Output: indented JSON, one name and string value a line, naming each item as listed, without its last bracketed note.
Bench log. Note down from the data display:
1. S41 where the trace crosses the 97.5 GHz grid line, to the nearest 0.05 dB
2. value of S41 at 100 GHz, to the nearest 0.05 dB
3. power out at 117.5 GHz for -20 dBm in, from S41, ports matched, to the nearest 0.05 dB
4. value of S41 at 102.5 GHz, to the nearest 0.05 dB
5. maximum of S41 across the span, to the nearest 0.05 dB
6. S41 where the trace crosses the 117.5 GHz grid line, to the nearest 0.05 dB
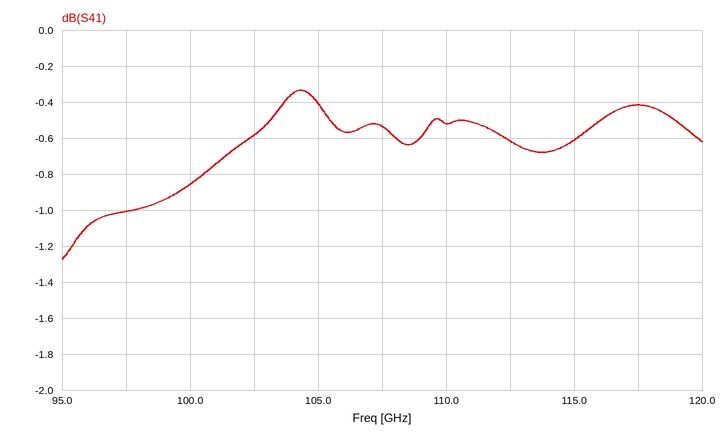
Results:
{
  "S41 where the trace crosses the 97.5 GHz grid line, to the nearest 0.05 dB": "-1.00 dB",
  "value of S41 at 100 GHz, to the nearest 0.05 dB": "-0.85 dB",
  "power out at 117.5 GHz for -20 dBm in, from S41, ports matched, to the nearest 0.05 dB": "-20.40 dBm",
  "value of S41 at 102.5 GHz, to the nearest 0.05 dB": "-0.60 dB",
  "maximum of S41 across the span, to the nearest 0.05 dB": "-0.35 dB",
  "S41 where the trace crosses the 117.5 GHz grid line, to the nearest 0.05 dB": "-0.40 dB"
}
